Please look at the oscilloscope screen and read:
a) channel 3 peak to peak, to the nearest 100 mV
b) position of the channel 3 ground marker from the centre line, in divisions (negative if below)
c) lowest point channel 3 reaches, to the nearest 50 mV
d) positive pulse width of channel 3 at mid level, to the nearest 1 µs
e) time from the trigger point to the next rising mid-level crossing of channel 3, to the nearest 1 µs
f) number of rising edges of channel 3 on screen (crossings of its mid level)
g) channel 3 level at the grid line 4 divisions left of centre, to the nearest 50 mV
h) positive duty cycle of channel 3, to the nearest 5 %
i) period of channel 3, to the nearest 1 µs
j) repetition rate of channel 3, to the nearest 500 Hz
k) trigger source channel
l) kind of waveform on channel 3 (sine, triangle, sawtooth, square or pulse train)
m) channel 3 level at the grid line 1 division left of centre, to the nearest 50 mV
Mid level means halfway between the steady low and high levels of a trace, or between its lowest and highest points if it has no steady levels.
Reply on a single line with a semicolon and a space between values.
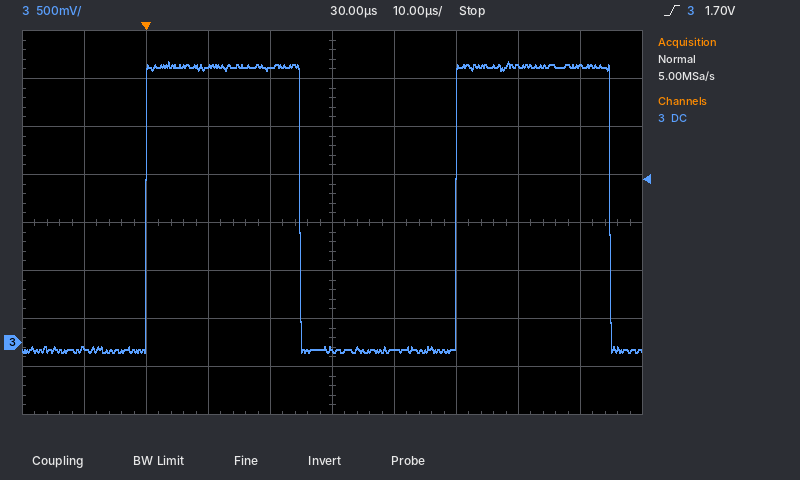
3.00 V; -2.5 div; -100 mV; 25 µs; 50 µs; 2; -50 mV; 50 %; 50 µs; 20.0 kHz; channel 3; square; 2.85 V
